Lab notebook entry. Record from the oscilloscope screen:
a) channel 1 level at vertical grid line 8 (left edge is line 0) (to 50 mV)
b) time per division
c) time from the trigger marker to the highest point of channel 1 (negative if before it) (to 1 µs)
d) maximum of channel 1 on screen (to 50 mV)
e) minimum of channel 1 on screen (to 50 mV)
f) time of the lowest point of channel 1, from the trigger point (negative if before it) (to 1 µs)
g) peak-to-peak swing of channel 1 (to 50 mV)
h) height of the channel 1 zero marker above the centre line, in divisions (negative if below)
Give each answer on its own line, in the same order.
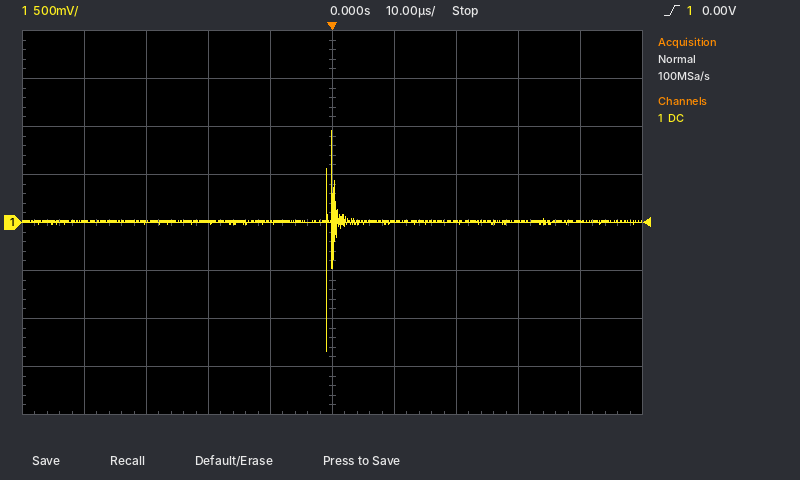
0 mV
10 µs
0 µs
950 mV
-1.35 V
-1 µs
2.30 V
0.0 div
